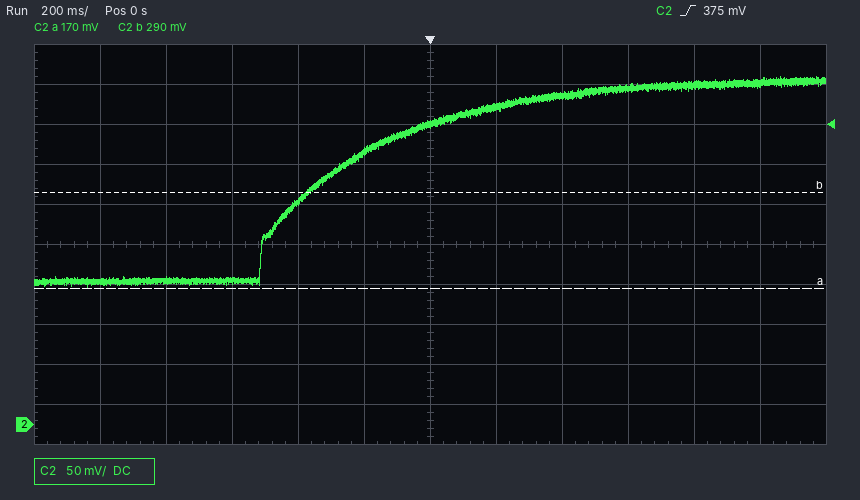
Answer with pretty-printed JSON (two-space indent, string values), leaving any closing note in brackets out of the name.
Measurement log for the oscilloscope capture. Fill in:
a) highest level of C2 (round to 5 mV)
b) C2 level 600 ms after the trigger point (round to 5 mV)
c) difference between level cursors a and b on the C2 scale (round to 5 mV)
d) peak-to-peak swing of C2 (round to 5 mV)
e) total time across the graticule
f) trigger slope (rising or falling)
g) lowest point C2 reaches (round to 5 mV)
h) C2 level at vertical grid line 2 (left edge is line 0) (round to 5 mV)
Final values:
{
  "highest level of C2": "435 mV",
  "C2 level 600 ms after the trigger point": "420 mV",
  "difference between level cursors a and b on the C2 scale": "120 mV",
  "peak-to-peak swing of C2": "265 mV",
  "total time across the graticule": "2.4 s",
  "trigger slope": "rising",
  "lowest point C2 reaches": "170 mV",
  "C2 level at vertical grid line 2 (left edge is line 0)": "180 mV"
}
